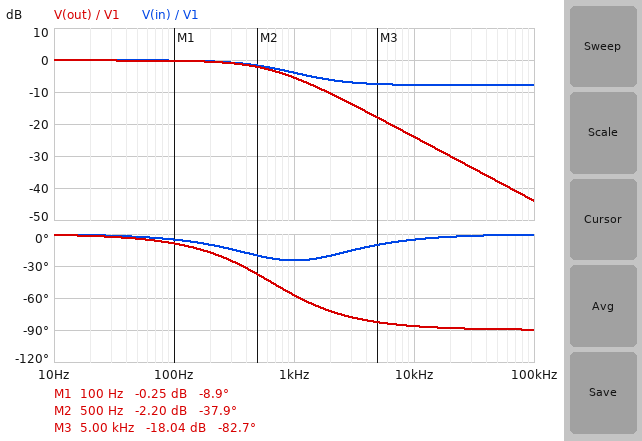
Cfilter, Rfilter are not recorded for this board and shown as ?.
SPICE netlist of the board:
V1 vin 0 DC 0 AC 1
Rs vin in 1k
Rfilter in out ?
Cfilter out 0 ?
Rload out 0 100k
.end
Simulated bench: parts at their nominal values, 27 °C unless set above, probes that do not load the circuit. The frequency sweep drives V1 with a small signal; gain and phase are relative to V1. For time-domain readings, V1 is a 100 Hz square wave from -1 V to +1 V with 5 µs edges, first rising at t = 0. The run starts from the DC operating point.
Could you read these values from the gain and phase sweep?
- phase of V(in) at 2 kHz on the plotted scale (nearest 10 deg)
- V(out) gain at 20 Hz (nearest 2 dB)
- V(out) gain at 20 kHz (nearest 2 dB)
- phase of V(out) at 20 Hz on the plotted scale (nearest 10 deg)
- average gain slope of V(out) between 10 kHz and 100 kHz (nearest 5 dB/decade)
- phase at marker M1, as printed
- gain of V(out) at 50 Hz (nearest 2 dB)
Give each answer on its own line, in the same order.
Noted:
-20 deg
0 dB
-30 dB
0 deg
-20 dB/decade
-8.9 deg
0 dB
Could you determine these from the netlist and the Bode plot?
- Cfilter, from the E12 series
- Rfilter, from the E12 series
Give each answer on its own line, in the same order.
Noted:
150 nF
680 Ω
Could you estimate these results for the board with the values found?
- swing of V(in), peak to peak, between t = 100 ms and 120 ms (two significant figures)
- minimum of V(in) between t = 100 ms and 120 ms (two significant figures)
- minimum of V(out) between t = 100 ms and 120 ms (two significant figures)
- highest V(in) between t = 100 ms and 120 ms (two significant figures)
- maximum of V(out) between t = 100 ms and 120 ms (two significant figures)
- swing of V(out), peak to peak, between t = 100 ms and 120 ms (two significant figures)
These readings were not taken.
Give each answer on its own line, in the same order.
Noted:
2.0 V
-990 mV
-980 mV
990 mV
980 mV
2.0 V
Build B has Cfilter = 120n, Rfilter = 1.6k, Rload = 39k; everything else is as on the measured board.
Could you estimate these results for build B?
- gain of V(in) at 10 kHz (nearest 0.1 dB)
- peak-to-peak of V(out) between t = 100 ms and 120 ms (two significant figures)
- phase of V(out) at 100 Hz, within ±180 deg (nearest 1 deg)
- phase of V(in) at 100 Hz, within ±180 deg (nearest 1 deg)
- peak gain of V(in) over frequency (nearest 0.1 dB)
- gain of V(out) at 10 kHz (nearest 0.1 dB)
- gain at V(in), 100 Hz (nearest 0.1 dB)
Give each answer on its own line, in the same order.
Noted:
-4.2 dB
1.9 V
-10 deg
-4 deg
-0.2 dB
-25.9 dB
-0.3 dB
